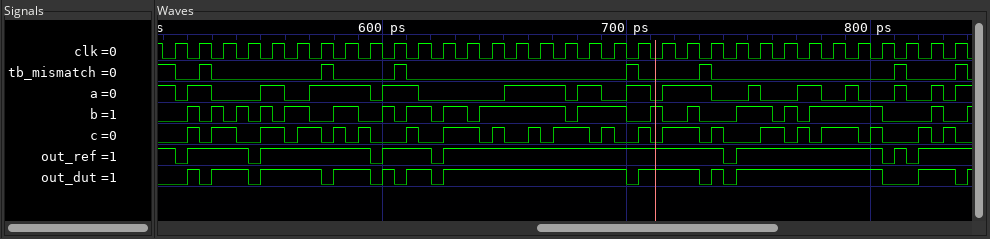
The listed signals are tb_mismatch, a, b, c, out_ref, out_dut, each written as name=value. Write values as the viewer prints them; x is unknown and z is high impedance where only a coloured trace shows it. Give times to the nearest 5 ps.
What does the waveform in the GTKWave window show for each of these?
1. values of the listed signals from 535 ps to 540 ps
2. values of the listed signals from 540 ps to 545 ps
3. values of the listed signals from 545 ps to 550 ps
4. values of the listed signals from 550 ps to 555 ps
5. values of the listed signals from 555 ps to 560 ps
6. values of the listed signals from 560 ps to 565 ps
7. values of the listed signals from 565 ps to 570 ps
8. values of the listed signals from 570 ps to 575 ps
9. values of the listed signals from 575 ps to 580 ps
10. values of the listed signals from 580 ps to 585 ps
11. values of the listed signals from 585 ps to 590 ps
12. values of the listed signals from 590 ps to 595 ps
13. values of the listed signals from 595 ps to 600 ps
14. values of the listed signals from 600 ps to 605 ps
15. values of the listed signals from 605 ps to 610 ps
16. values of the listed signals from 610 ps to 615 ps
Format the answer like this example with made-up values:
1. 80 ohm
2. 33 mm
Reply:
1. tb_mismatch=0, a=0, b=0, c=1, out_ref=1, out_dut=1
2. tb_mismatch=0, a=0, b=1, c=0, out_ref=1, out_dut=1
3. tb_mismatch=0, a=0, b=0, c=0, out_ref=0, out_dut=0
4. tb_mismatch=0, a=1, b=1, c=1, out_ref=1, out_dut=1
5. tb_mismatch=0, a=1, b=0, c=1, out_ref=1, out_dut=1
6. tb_mismatch=0, a=0, b=1, c=0, out_ref=1, out_dut=1
7. tb_mismatch=0, a=0, b=1, c=1, out_ref=1, out_dut=1
8. tb_mismatch=0, a=1, b=0, c=1, out_ref=1, out_dut=1
9. tb_mismatch=1, a=1, b=0, c=0, out_ref=1, out_dut=0
10. tb_mismatch=0, a=1, b=1, c=1, out_ref=1, out_dut=1
11. tb_mismatch=0, a=1, b=1, c=0, out_ref=1, out_dut=1
12. tb_mismatch=0, a=1, b=0, c=1, out_ref=1, out_dut=1
13. tb_mismatch=0, a=0, b=0, c=0, out_ref=0, out_dut=0
14. tb_mismatch=0, a=1, b=1, c=0, out_ref=1, out_dut=1
15. tb_mismatch=1, a=1, b=0, c=0, out_ref=1, out_dut=0
16. tb_mismatch=0, a=1, b=1, c=1, out_ref=1, out_dut=1
